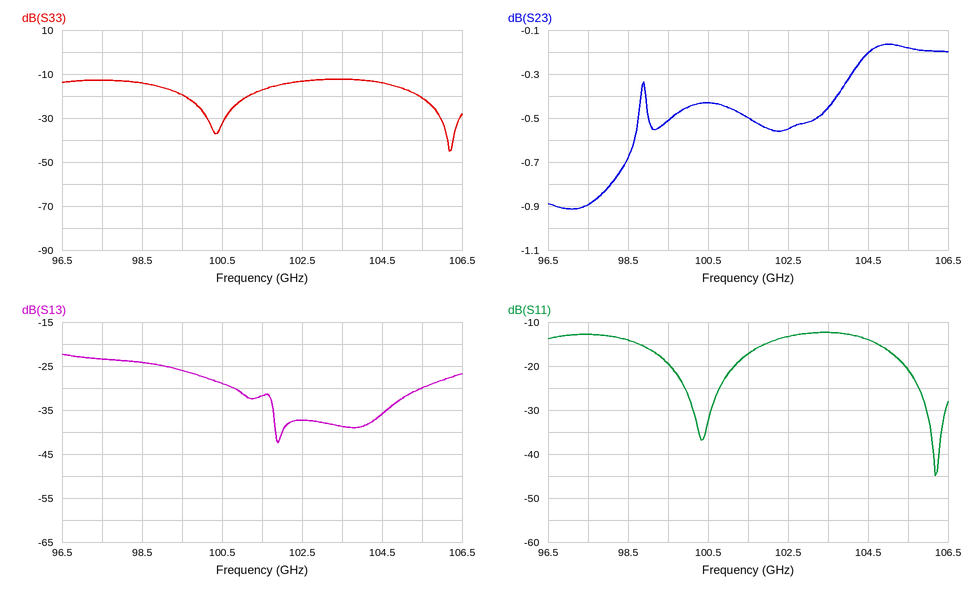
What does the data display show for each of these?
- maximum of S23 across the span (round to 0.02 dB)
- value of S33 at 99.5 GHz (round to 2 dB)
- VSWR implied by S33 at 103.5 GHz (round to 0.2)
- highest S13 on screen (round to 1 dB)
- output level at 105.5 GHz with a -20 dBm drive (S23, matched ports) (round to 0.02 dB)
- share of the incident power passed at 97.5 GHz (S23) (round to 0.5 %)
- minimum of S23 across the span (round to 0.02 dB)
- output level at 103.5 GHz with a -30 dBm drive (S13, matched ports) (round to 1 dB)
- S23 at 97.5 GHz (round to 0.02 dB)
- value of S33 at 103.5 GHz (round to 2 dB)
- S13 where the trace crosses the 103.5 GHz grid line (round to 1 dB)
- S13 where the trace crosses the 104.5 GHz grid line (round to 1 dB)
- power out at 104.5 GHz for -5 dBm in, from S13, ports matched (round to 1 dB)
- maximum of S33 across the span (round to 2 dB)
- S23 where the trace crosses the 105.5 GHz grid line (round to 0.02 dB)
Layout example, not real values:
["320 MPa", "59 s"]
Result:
["-0.16 dB", "-20 dB", "1.6", "-22 dB", "-20.18 dBm", "81.5 %", "-0.92 dB", "-69 dBm", "-0.90 dB", "-12 dB", "-39 dB", "-36 dB", "-41 dBm", "-12 dB", "-0.18 dB"]
